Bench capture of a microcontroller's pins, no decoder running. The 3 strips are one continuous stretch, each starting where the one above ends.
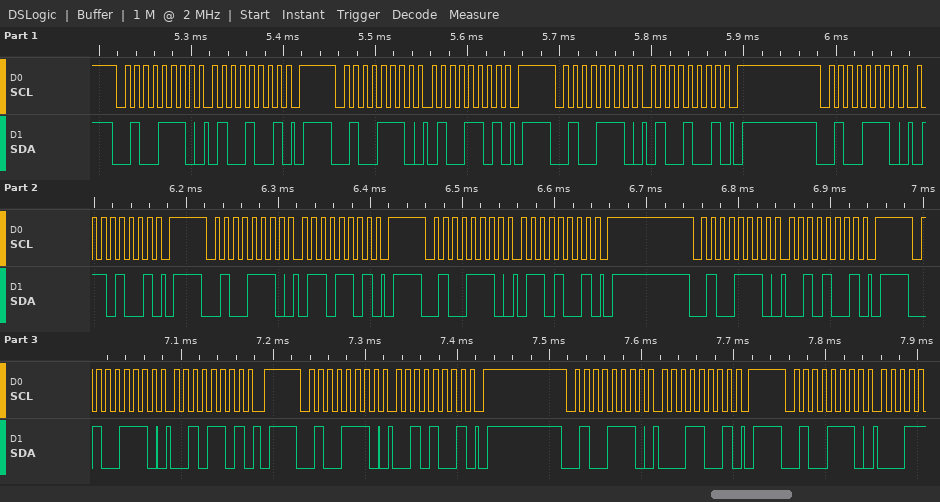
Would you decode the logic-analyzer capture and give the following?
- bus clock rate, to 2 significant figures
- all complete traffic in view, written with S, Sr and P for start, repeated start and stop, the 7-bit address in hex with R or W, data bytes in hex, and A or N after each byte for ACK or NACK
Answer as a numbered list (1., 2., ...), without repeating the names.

1. 100 kHz
2. S 27W A 49 A P S 27W A 4D A P S 27W A 49 A P S 27W A 69 A P S 27W A 6D A P S 27W A 69 A P S 27W A 29 A P S 27W A 2D A P S 27W A 29 A P S 27W A 19 A P S 27W A
